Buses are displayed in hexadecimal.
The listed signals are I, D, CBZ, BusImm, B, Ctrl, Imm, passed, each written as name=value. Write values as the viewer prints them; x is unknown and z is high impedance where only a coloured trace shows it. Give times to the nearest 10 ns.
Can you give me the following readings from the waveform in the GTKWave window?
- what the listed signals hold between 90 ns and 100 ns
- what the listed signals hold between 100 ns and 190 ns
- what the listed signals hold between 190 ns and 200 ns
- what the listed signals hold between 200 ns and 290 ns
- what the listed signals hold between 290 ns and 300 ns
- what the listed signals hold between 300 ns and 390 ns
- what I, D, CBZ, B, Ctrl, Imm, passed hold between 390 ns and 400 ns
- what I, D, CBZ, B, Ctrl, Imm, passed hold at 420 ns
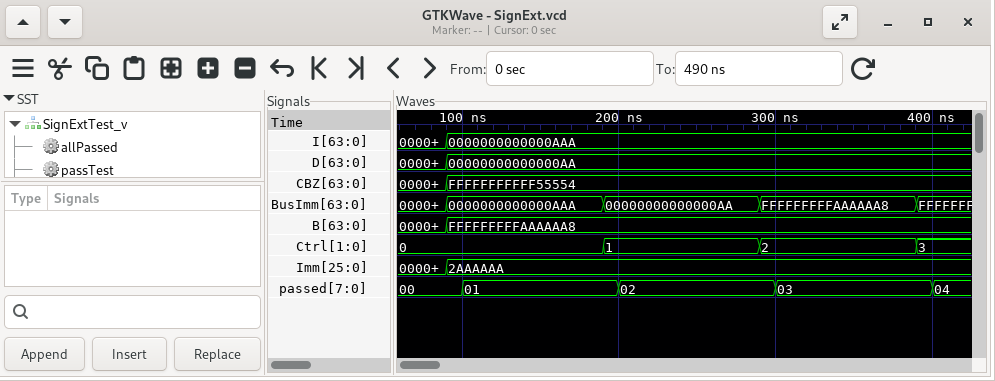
I=0000000000000AAA, D=00000000000000AA, CBZ=FFFFFFFFFFF55554, BusImm=0000000000000AAA, B=FFFFFFFFFAAAAAA8, Ctrl=0, Imm=2AAAAAA, passed=00
I=0000000000000AAA, D=00000000000000AA, CBZ=FFFFFFFFFFF55554, BusImm=0000000000000AAA, B=FFFFFFFFFAAAAAA8, Ctrl=0, Imm=2AAAAAA, passed=01
I=0000000000000AAA, D=00000000000000AA, CBZ=FFFFFFFFFFF55554, BusImm=00000000000000AA, B=FFFFFFFFFAAAAAA8, Ctrl=1, Imm=2AAAAAA, passed=01
I=0000000000000AAA, D=00000000000000AA, CBZ=FFFFFFFFFFF55554, BusImm=00000000000000AA, B=FFFFFFFFFAAAAAA8, Ctrl=1, Imm=2AAAAAA, passed=02
I=0000000000000AAA, D=00000000000000AA, CBZ=FFFFFFFFFFF55554, BusImm=FFFFFFFFFAAAAAA8, B=FFFFFFFFFAAAAAA8, Ctrl=2, Imm=2AAAAAA, passed=02
I=0000000000000AAA, D=00000000000000AA, CBZ=FFFFFFFFFFF55554, BusImm=FFFFFFFFFAAAAAA8, B=FFFFFFFFFAAAAAA8, Ctrl=2, Imm=2AAAAAA, passed=03
I=0000000000000AAA, D=00000000000000AA, CBZ=FFFFFFFFFFF55554, B=FFFFFFFFFAAAAAA8, Ctrl=3, Imm=2AAAAAA, passed=03
I=0000000000000AAA, D=00000000000000AA, CBZ=FFFFFFFFFFF55554, B=FFFFFFFFFAAAAAA8, Ctrl=3, Imm=2AAAAAA, passed=04
